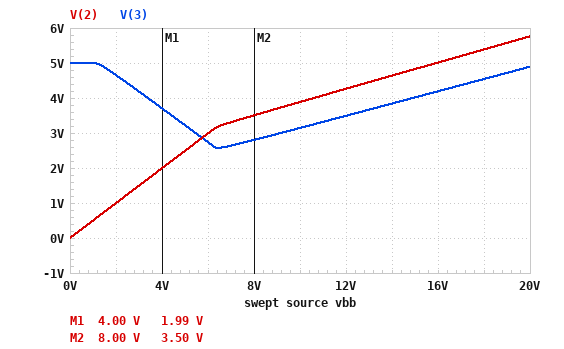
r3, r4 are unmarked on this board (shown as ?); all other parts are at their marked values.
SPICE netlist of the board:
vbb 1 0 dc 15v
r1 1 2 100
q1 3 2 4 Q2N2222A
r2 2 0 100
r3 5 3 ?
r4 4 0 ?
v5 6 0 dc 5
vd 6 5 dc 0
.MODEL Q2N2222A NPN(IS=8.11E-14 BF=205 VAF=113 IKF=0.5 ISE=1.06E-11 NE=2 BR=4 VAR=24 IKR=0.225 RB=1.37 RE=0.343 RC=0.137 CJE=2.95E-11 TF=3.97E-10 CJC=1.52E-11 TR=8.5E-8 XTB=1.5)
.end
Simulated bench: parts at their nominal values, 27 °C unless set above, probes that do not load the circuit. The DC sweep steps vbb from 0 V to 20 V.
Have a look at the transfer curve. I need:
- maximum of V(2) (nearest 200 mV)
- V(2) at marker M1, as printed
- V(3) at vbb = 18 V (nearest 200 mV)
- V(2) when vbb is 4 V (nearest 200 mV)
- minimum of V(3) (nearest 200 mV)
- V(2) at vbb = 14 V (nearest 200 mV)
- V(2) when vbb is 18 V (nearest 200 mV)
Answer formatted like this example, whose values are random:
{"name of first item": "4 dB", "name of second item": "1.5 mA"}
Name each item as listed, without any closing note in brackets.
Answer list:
{"maximum of V(2)": "5.8 V", "V(2) at marker M1, as printed": "1.99 V", "V(3) at vbb = 18 V": "4.6 V", "V(2) when vbb is 4 V": "2.0 V", "minimum of V(3)": "2.6 V", "V(2) at vbb = 14 V": "4.6 V", "V(2) when vbb is 18 V": "5.4 V"}
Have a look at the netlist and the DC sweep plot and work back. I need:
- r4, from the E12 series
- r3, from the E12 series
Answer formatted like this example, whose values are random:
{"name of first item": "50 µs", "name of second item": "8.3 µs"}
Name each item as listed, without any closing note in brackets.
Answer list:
{"r4, from the E12 series": "56 Ω", "r3, from the E12 series": "56 Ω"}
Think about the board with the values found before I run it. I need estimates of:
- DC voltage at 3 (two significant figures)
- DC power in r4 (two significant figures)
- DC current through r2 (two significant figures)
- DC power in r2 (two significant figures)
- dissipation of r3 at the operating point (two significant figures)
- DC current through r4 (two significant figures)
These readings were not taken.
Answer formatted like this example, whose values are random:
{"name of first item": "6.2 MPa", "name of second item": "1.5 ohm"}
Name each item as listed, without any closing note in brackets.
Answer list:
{"DC voltage at 3": "4.0 V", "DC power in r4": "280 mW", "DC current through r2": "48 mA", "DC power in r2": "230 mW", "dissipation of r3 at the operating point": "17 mW", "DC current through r4": "71 mA"}
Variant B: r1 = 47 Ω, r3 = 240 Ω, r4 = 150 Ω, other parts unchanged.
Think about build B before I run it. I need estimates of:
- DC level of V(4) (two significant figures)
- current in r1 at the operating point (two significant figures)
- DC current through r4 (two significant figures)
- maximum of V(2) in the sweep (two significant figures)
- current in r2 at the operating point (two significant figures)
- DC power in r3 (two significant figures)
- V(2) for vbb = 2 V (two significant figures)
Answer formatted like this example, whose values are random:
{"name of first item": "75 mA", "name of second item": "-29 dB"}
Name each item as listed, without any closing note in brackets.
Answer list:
{"DC level of V(4)": "7.4 V", "current in r1 at the operating point": "140 mA", "DC current through r4": "50 mA", "maximum of V(2) in the sweep": "11 V", "current in r2 at the operating point": "83 mA", "DC power in r3": "25 mW", "V(2) for vbb = 2 V": "1.4 V"}
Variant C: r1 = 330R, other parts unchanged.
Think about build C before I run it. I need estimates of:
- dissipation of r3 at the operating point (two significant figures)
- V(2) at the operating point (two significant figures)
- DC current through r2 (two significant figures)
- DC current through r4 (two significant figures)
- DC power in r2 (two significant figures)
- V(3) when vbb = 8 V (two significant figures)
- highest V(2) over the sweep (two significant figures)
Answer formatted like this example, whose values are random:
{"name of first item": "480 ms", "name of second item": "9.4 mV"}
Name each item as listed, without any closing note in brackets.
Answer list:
{"dissipation of r3 at the operating point": "100 mW", "V(2) at the operating point": "3.3 V", "DC current through r2": "33 mA", "DC current through r4": "45 mA", "DC power in r2": "110 mW", "V(3) when vbb = 8 V": "3.8 V", "highest V(2) over the sweep": "3.6 V"}
